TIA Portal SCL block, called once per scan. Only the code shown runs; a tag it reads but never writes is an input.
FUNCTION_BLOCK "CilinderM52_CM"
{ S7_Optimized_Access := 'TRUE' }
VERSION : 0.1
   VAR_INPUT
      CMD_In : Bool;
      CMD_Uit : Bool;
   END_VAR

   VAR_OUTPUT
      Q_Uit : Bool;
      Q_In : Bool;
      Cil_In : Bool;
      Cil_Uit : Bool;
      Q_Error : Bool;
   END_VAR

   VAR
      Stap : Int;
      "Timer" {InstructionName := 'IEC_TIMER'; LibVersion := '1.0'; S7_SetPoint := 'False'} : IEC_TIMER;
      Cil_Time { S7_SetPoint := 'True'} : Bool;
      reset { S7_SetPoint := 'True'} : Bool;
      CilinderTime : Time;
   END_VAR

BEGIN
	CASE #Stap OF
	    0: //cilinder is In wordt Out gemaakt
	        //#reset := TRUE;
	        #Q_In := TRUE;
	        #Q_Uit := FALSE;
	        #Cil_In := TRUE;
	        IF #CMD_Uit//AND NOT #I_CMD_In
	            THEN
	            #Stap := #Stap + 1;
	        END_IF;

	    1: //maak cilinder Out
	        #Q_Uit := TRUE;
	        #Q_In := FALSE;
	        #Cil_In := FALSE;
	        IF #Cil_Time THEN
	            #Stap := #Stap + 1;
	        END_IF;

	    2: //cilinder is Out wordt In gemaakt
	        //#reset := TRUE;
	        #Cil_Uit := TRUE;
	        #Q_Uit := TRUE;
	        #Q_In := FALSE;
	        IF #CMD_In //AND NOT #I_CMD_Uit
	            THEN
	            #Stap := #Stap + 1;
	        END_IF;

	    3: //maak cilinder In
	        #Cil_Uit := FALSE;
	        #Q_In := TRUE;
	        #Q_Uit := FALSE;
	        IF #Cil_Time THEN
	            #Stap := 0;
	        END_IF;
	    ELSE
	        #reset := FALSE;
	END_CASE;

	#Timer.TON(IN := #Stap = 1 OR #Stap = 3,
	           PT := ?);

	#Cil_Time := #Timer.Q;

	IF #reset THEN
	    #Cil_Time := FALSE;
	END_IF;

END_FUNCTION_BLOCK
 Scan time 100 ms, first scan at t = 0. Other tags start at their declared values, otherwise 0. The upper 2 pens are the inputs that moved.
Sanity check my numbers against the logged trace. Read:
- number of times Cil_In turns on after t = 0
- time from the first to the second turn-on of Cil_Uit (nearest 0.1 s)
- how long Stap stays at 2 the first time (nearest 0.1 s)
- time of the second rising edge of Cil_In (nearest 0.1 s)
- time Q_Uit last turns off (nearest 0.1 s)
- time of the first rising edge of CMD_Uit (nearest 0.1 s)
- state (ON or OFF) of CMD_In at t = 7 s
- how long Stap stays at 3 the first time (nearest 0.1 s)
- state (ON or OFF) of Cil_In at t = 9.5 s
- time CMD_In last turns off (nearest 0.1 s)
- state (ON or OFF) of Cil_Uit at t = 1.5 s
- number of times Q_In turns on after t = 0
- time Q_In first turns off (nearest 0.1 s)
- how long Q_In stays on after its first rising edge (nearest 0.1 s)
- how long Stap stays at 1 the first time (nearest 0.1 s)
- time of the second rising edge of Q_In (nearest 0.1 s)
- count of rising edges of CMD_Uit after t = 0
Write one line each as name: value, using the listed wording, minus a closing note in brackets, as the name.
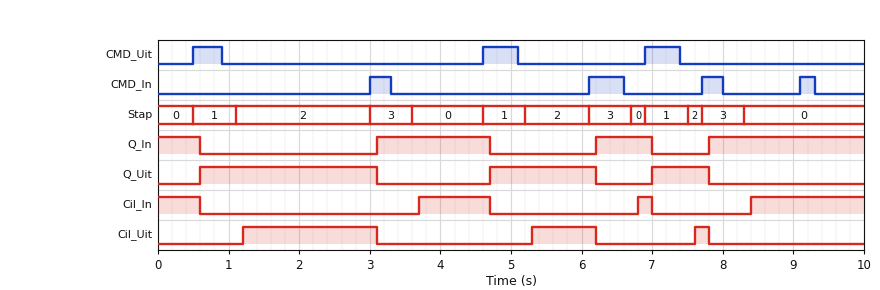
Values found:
number of times Cil_In turns on after t = 0: 3
time from the first to the second turn-on of Cil_Uit: 4.1 s
how long Stap stays at 2 the first time: 1.9 s
time of the second rising edge of Cil_In: 6.8 s
time Q_Uit last turns off: 7.8 s
time of the first rising edge of CMD_Uit: 0.5 s
state (ON or OFF) of CMD_In at t = 7 s: OFF
how long Stap stays at 3 the first time: 0.6 s
state (ON or OFF) of Cil_In at t = 9.5 s: ON
time CMD_In last turns off: 9.3 s
state (ON or OFF) of Cil_Uit at t = 1.5 s: ON
number of times Q_In turns on after t = 0: 3
time Q_In first turns off: 0.6 s
how long Q_In stays on after its first rising edge: 1.6 s
how long Stap stays at 1 the first time: 0.6 s
time of the second rising edge of Q_In: 6.2 s
count of rising edges of CMD_Uit after t = 0: 3
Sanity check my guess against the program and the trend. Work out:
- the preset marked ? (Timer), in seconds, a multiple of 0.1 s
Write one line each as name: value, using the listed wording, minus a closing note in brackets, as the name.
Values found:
the preset marked ? (Timer), in seconds, a multiple of 0.1 s: 0.5 s
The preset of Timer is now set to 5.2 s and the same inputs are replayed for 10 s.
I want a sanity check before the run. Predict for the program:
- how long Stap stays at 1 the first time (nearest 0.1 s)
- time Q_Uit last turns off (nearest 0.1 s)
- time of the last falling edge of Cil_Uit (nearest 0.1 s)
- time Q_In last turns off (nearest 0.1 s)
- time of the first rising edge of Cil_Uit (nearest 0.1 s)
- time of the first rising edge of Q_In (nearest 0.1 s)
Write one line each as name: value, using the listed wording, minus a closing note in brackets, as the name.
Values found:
how long Stap stays at 1 the first time: 5.3 s
time Q_Uit last turns off: 6.2 s
time of the last falling edge of Cil_Uit: 6.2 s
time Q_In last turns off: 0.6 s
time of the first rising edge of Cil_Uit: 5.9 s
time of the first rising edge of Q_In: 6.2 s
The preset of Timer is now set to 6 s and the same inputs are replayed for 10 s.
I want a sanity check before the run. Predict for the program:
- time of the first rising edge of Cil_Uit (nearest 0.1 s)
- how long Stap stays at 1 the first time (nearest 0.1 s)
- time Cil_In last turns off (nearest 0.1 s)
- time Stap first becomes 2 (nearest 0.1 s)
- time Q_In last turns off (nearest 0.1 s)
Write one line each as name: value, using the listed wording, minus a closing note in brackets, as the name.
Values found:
time of the first rising edge of Cil_Uit: 6.7 s
how long Stap stays at 1 the first time: 6.1 s
time Cil_In last turns off: 0.6 s
time Stap first becomes 2: 6.6 s
time Q_In last turns off: 0.6 s
